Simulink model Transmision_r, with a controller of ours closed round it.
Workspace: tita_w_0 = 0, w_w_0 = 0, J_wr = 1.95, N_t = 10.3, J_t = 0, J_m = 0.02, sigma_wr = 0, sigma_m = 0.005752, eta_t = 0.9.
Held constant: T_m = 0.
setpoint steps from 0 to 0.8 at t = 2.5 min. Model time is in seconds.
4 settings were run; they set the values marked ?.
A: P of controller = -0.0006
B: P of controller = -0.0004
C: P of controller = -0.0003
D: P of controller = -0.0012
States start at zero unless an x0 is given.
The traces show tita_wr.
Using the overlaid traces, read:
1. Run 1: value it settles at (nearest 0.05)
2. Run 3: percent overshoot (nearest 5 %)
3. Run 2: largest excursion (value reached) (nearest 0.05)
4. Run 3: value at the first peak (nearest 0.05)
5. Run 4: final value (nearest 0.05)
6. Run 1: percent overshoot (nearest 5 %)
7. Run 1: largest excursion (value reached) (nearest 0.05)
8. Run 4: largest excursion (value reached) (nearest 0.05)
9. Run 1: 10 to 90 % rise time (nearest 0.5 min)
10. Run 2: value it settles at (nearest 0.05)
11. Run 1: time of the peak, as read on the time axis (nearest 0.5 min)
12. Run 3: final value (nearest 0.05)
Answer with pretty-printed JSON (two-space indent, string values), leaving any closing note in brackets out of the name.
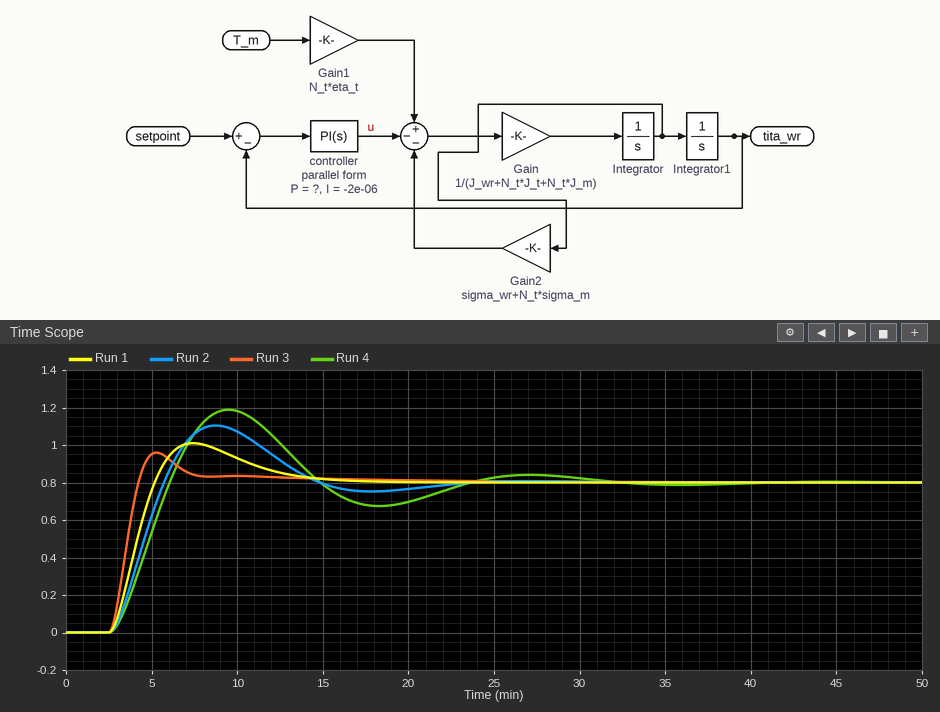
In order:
{
  "Run 1: value it settles at": "0.80",
  "Run 3: percent overshoot": "20 %",
  "Run 2: largest excursion (value reached)": "1.10",
  "Run 3: value at the first peak": "0.95",
  "Run 4: final value": "0.80",
  "Run 1: percent overshoot": "25 %",
  "Run 1: largest excursion (value reached)": "1.00",
  "Run 4: largest excursion (value reached)": "1.20",
  "Run 1: 10 to 90 % rise time": "2.0 min",
  "Run 2: value it settles at": "0.80",
  "Run 1: time of the peak, as read on the time axis": "7.5 min",
  "Run 3: final value": "0.80"
}
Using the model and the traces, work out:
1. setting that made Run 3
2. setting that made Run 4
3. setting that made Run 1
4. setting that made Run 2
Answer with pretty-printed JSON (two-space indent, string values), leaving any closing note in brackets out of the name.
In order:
{
  "setting that made Run 3": "D",
  "setting that made Run 4": "C",
  "setting that made Run 1": "A",
  "setting that made Run 2": "B"
}
